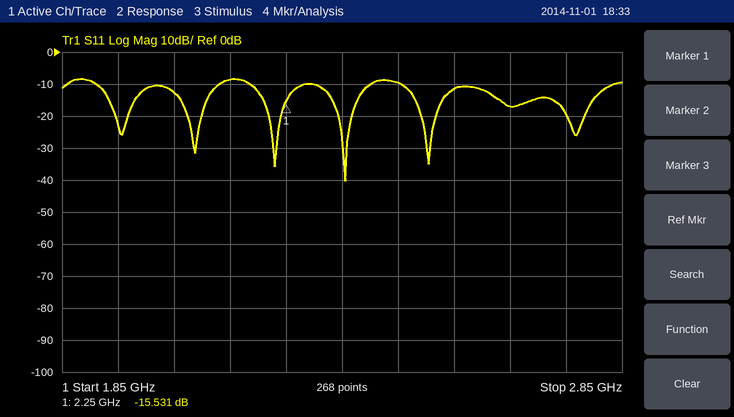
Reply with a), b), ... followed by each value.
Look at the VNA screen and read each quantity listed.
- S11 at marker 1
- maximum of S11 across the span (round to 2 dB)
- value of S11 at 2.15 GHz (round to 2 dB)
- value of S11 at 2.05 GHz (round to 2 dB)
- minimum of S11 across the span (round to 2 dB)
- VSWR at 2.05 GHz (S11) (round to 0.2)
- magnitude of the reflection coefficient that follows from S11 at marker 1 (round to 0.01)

a) -15.531 dB
b) -8 dB
c) -8 dB
d) -12 dB
e) -40 dB
f) 1.6
g) 0.17
